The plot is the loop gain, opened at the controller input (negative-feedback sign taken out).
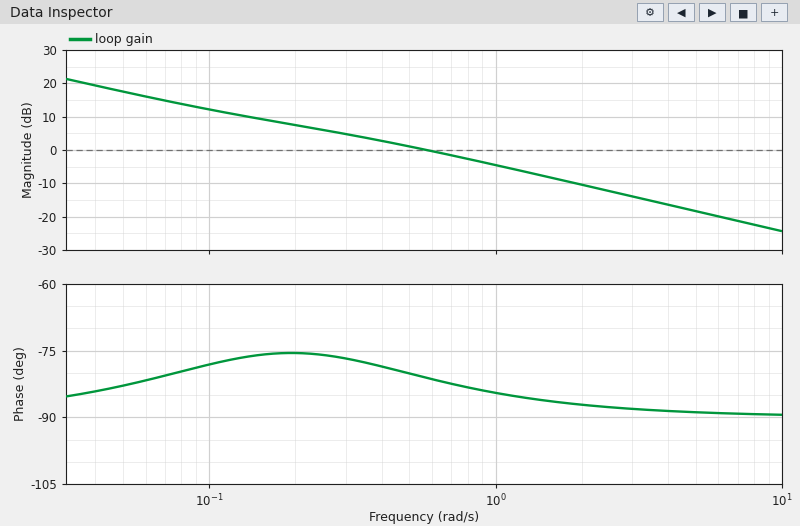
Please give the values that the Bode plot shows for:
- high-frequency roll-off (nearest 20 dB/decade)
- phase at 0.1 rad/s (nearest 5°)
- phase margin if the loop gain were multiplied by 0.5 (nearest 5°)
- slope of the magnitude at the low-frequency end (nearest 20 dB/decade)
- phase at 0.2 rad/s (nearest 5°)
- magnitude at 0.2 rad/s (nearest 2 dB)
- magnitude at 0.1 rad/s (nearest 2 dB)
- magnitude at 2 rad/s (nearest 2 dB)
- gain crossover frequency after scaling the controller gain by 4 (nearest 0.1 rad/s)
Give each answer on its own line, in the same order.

-20 dB/decade
-80°
105°
-20 dB/decade
-75°
8 dB
12 dB
-10 dB
2.4 rad/s
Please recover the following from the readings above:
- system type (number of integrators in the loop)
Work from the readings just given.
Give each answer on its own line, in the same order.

1
